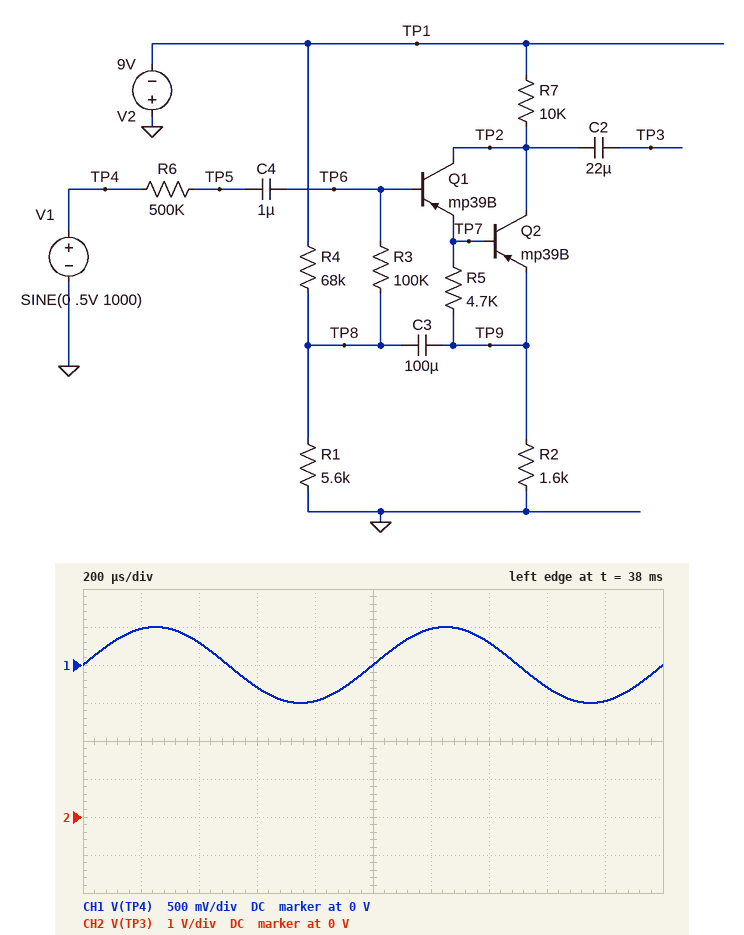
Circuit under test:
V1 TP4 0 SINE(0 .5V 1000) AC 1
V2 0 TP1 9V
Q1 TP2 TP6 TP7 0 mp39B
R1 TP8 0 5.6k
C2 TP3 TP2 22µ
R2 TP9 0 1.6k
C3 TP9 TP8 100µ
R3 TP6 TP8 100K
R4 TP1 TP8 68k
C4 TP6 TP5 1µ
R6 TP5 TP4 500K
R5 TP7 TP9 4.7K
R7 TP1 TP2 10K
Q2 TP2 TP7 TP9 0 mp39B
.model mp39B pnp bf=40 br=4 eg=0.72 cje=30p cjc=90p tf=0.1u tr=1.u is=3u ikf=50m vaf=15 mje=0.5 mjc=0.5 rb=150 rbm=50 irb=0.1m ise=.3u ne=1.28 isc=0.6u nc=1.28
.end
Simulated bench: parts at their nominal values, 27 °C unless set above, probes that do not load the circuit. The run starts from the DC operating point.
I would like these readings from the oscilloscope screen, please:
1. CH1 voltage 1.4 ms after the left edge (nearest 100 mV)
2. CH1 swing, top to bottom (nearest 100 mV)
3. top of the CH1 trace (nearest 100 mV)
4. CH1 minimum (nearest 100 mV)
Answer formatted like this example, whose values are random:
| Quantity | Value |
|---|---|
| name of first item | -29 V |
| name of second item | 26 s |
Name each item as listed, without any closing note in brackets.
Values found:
| Quantity | Value |
|---|---|
| CH1 voltage 1.4 ms after the left edge | 300 mV |
| CH1 swing, top to bottom | 1.0 V |
| top of the CH1 trace | 500 mV |
| CH1 minimum | -500 mV |
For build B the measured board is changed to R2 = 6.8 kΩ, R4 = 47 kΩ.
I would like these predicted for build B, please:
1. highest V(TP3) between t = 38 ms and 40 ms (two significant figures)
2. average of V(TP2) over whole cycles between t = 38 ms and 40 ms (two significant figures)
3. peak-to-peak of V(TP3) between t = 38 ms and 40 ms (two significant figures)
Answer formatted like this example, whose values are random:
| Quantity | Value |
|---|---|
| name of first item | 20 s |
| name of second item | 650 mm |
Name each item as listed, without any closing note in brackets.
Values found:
| Quantity | Value |
|---|---|
| highest V(TP3) between t = 38 ms and 40 ms | -8.5 V |
| average of V(TP2) over whole cycles between t = 38 ms and 40 ms | -8.7 V |
| peak-to-peak of V(TP3) between t = 38 ms and 40 ms | 380 mV |
